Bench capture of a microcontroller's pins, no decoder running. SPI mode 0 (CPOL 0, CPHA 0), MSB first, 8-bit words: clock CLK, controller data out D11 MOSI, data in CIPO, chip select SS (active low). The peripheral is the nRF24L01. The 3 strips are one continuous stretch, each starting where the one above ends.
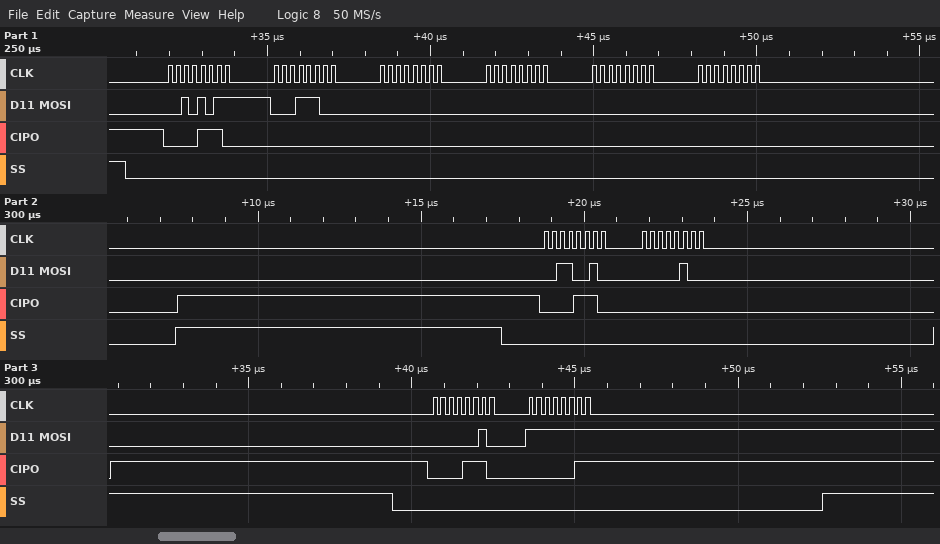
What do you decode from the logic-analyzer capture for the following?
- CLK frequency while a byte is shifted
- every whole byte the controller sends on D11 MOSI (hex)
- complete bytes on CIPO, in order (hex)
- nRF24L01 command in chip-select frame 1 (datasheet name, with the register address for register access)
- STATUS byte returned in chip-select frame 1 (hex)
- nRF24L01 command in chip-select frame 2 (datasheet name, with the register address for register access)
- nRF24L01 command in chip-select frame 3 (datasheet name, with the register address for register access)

4 MHz
2B 1C 00 00 00 00 32 04 02 FF
0E 00 00 00 00 00 0E 00 0E 03
W_REGISTER 0x0B
0x0E
W_REGISTER 0x12
R_REGISTER 0x02
